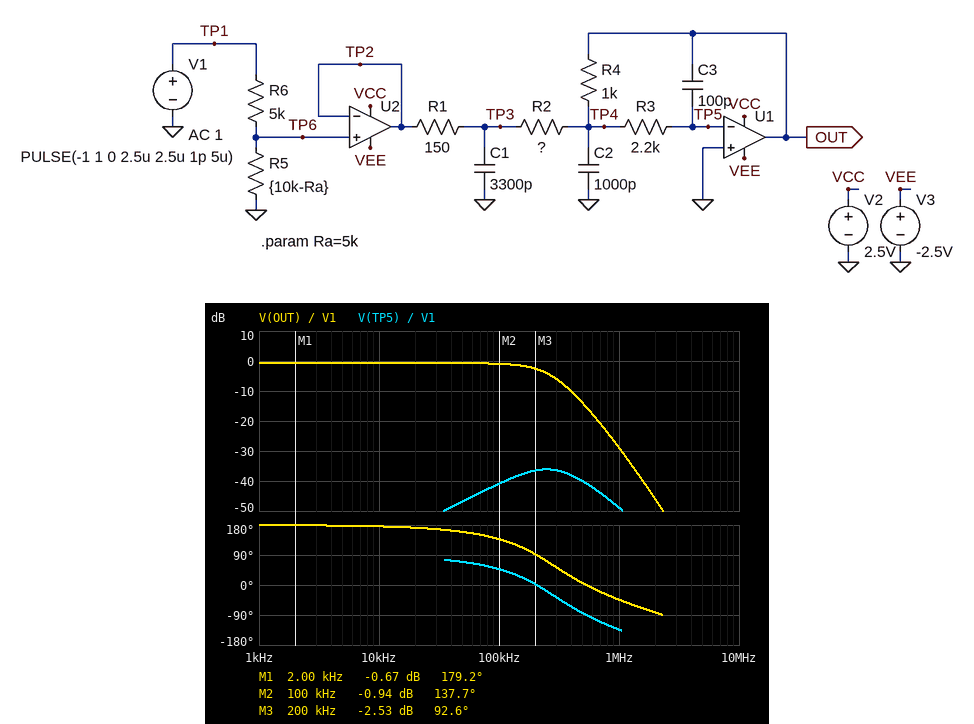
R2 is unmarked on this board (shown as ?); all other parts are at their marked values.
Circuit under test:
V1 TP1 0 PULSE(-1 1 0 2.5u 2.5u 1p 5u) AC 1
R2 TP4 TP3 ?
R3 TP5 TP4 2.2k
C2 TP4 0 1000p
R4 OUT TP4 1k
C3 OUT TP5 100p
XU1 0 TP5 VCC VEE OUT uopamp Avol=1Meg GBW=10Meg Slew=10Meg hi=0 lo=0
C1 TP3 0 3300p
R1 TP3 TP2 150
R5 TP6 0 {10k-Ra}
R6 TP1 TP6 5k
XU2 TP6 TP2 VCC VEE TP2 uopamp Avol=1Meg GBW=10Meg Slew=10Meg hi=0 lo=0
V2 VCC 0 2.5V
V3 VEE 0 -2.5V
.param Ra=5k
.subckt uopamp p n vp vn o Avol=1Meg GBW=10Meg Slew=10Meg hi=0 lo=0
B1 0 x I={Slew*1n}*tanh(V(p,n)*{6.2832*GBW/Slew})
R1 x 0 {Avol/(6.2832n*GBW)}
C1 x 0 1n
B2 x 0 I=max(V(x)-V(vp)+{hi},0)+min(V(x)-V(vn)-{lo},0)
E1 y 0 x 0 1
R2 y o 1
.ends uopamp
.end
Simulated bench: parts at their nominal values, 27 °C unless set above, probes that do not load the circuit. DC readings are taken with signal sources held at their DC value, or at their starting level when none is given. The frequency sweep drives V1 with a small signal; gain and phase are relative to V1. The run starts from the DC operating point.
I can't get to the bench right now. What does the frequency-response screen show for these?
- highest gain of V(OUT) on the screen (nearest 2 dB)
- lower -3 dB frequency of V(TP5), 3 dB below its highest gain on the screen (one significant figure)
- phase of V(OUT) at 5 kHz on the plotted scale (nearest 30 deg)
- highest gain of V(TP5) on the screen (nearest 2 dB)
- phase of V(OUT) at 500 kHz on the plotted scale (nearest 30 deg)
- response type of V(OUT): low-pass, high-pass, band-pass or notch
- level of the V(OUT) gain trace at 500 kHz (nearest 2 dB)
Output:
0 dB
100 kHz
180 deg
-36 dB
0 deg
low-pass
-14 dB
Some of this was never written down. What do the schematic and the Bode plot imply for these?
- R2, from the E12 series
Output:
390 Ω
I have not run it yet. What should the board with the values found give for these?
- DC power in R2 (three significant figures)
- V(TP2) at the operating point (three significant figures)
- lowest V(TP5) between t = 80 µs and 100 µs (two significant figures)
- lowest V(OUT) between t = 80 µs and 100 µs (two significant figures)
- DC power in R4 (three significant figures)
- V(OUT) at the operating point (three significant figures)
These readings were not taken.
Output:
334 µW
-500 mV
-12 mV
-610 mV
857 µW
926 mV
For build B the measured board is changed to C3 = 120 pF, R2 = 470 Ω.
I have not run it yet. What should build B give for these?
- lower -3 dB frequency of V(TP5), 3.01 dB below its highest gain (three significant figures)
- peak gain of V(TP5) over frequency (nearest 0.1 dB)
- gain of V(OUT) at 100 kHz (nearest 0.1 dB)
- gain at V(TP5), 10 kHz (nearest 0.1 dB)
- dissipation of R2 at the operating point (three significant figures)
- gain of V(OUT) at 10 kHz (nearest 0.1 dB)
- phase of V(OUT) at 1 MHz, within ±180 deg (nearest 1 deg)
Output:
118 kHz
-38.0 dB
-2.3 dB
-61.9 dB
306 µW
-1.9 dB
-48 deg
